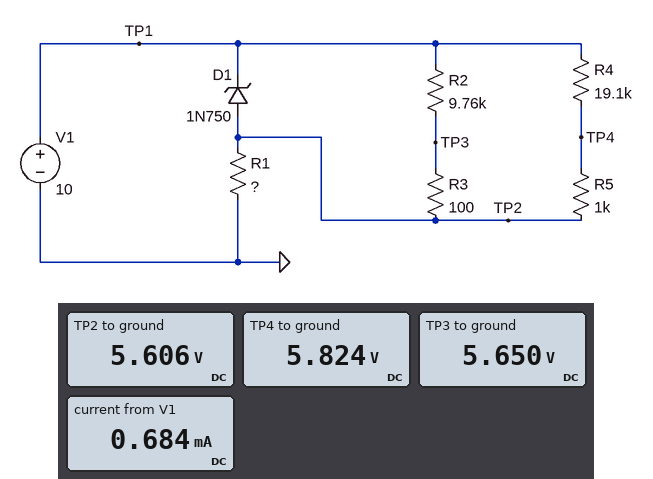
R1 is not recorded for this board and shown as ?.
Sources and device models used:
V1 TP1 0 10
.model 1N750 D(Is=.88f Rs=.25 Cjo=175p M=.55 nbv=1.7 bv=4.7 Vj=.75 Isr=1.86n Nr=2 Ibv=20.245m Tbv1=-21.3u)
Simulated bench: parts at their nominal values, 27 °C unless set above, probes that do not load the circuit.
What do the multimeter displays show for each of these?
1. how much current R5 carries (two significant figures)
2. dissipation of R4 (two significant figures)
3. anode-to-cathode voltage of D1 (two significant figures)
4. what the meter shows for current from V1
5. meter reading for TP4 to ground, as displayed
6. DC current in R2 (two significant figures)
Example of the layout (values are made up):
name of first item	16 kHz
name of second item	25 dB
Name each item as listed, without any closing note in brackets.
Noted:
how much current R5 carries	220 µA
dissipation of R4	910 µW
anode-to-cathode voltage of D1	-4.4 V
what the meter shows for current from V1	0.684 mA
meter reading for TP4 to ground, as displayed	5.824 V
DC current in R2	450 µA
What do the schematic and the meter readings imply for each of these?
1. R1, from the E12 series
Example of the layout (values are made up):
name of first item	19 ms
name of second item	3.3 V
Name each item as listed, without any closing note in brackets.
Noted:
R1, from the E12 series	8.2 kΩ
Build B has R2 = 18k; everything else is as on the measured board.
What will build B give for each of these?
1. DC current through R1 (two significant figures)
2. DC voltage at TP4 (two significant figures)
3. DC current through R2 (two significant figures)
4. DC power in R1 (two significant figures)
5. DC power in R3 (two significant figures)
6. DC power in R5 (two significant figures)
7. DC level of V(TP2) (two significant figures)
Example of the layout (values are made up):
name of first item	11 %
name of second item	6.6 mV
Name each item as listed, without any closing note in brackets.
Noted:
DC current through R1	670 µA
DC voltage at TP4	5.7 V
DC current through R2	250 µA
DC power in R1	3.7 mW
DC power in R3	6.2 µW
DC power in R5	50 µW
DC level of V(TP2)	5.5 V
